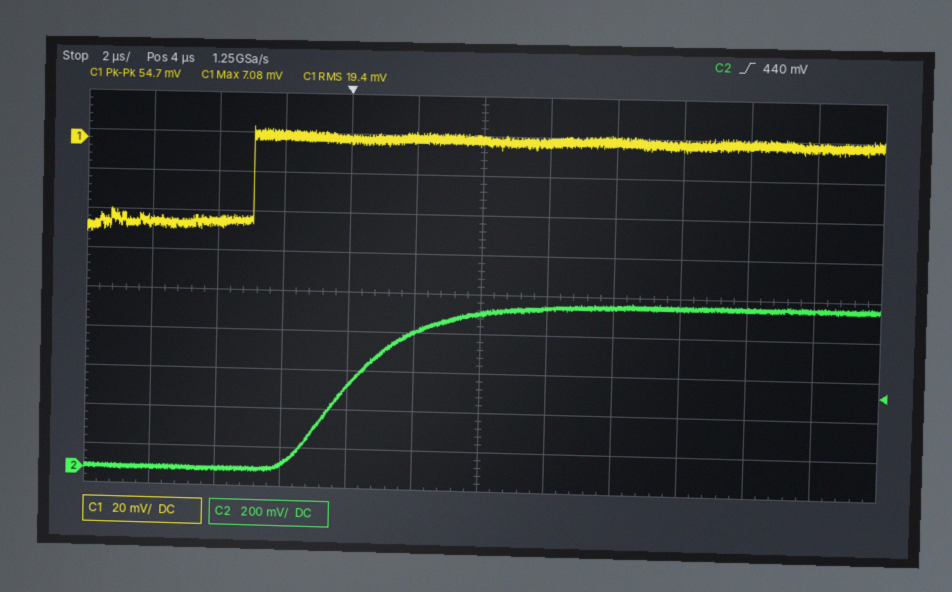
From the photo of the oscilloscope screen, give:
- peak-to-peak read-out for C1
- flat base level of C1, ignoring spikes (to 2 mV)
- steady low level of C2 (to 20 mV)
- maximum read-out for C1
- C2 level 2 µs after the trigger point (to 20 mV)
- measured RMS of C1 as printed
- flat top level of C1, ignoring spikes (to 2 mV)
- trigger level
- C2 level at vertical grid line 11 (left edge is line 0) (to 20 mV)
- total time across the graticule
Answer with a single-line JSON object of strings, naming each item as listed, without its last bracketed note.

{"peak-to-peak read-out for C1": "54.7 mV", "flat base level of C1, ignoring spikes": "-42 mV", "steady low level of C2": "0 mV", "maximum read-out for C1": "7.08 mV", "C2 level 2 µs after the trigger point": "720 mV", "measured RMS of C1 as printed": "19.4 mV", "flat top level of C1, ignoring spikes": "2 mV", "trigger level": "440 mV", "C2 level at vertical grid line 11 (left edge is line 0)": "880 mV", "total time across the graticule": "24 µs"}
